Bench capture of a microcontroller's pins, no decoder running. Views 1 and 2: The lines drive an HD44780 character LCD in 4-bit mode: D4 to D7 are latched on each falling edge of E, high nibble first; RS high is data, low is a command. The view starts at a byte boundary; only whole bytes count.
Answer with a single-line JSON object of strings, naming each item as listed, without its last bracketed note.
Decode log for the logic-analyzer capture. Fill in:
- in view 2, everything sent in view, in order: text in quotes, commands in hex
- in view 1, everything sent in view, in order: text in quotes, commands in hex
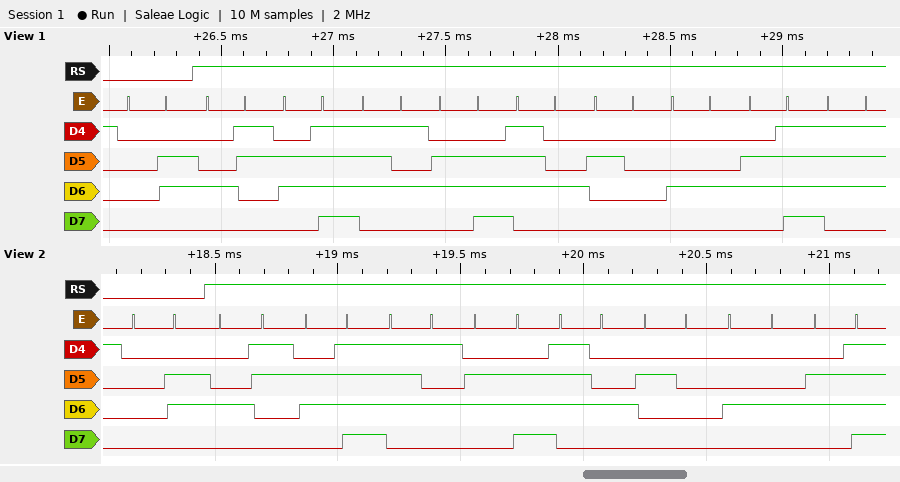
{"in view 2, everything sent in view, in order: text in quotes, commands in hex": "0x06 \"Count Do\"", "in view 1, everything sent in view, in order: text in quotes, commands in hex": "0x06 \"Count Dow\""}
